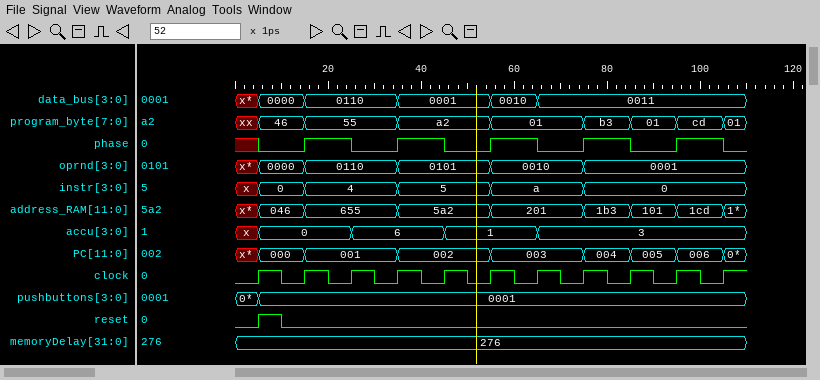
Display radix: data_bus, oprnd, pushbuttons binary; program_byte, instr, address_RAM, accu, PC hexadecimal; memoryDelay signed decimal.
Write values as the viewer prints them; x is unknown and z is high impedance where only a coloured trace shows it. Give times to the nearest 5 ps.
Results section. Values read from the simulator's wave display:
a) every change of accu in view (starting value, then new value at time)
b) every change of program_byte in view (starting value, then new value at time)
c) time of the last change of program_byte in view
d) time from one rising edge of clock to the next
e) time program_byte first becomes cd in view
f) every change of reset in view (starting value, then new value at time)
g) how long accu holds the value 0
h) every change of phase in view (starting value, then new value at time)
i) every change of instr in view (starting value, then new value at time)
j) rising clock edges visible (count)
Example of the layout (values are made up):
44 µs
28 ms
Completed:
x, 0 at 5 ps, 6 at 25 ps, 1 at 45 ps, 3 at 65 ps
xx, 46 at 5 ps, 55 at 15 ps, a2 at 35 ps, 01 at 55 ps, b3 at 75 ps, 01 at 85 ps, cd at 95 ps, 01 at 105 ps
105 ps
10 ps
95 ps
0, 1 at 5 ps, 0 at 10 ps
20 ps
x, 0 at 5 ps, 1 at 15 ps, 0 at 25 ps, 1 at 35 ps, 0 at 45 ps, 1 at 55 ps, 0 at 65 ps, 1 at 75 ps, 0 at 85 ps, 1 at 95 ps, 0 at 105 ps
x, 0 at 5 ps, 4 at 15 ps, 5 at 35 ps, a at 55 ps, 0 at 75 ps
11
